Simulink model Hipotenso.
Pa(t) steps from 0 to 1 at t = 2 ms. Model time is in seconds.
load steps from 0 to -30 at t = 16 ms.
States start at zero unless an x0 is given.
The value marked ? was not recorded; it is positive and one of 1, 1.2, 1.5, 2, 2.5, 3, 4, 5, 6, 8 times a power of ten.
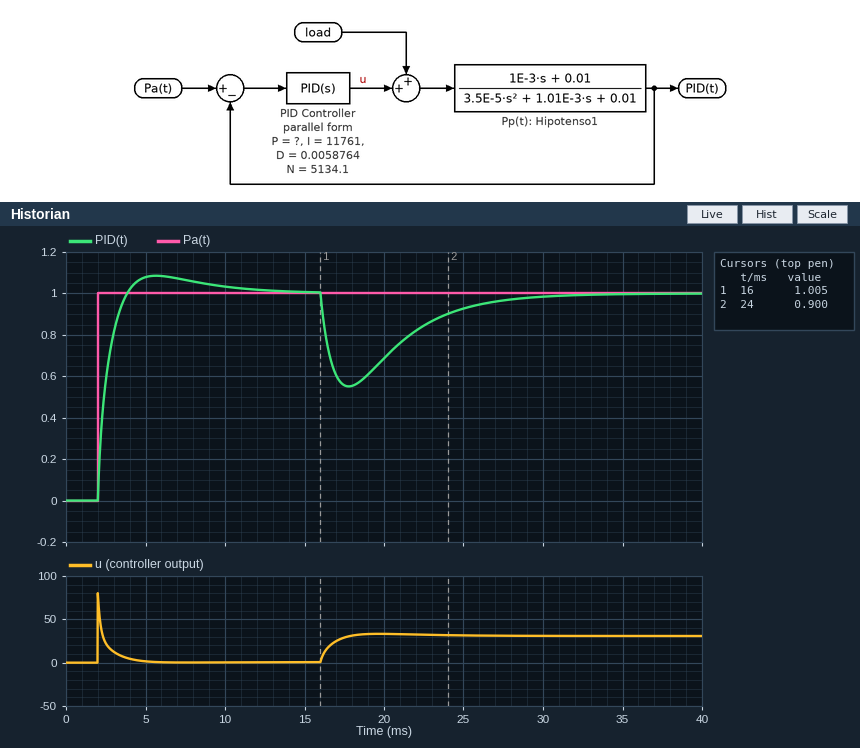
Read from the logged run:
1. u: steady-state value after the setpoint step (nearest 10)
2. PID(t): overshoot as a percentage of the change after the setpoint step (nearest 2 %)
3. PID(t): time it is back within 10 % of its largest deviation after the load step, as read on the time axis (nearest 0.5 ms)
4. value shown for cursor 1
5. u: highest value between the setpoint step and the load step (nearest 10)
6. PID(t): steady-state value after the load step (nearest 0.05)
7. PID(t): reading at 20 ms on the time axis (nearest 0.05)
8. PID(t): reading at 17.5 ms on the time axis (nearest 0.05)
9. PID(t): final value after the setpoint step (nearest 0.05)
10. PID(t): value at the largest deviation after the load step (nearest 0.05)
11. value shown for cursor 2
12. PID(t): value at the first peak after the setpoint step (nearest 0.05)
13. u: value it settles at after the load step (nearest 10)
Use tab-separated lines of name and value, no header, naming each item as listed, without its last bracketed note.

u: steady-state value after the setpoint step	0
PID(t): overshoot as a percentage of the change after the setpoint step	8 %
PID(t): time it is back within 10 % of its largest deviation after the load step, as read on the time axis	26.5 ms
value shown for cursor 1	1.005
u: highest value between the setpoint step and the load step	80
PID(t): steady-state value after the load step	1.00
PID(t): reading at 20 ms on the time axis	0.70
PID(t): reading at 17.5 ms on the time axis	0.55
PID(t): final value after the setpoint step	1.00
PID(t): value at the largest deviation after the load step	0.55
value shown for cursor 2	0.900
PID(t): value at the first peak after the setpoint step	1.10
u: value it settles at after the load step	30
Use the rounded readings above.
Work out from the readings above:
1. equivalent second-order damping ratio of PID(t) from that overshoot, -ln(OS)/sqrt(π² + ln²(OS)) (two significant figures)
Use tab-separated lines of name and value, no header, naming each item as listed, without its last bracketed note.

equivalent second-order damping ratio of PID(t) from that overshoot, -ln(OS)/sqrt(π² + ln²(OS))	0.63
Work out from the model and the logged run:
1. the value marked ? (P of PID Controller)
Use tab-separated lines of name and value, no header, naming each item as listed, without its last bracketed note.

the value marked ?	50
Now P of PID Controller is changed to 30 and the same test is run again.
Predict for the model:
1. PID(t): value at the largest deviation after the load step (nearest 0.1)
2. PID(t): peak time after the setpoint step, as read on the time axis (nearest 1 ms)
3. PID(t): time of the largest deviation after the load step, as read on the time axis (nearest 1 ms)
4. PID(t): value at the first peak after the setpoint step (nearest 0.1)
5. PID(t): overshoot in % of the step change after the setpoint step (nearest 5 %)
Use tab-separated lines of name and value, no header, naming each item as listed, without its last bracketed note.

PID(t): value at the largest deviation after the load step	0.4
PID(t): peak time after the setpoint step, as read on the time axis	6 ms
PID(t): time of the largest deviation after the load step, as read on the time axis	18 ms
PID(t): value at the first peak after the setpoint step	1.2
PID(t): overshoot in % of the step change after the setpoint step	15 %
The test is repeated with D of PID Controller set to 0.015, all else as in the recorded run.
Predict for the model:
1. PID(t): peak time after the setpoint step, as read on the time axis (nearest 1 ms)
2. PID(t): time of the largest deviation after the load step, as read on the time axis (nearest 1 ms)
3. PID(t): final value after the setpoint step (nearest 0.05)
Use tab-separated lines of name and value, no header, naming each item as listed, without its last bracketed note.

PID(t): peak time after the setpoint step, as read on the time axis	6 ms
PID(t): time of the largest deviation after the load step, as read on the time axis	18 ms
PID(t): final value after the setpoint step	1.00
